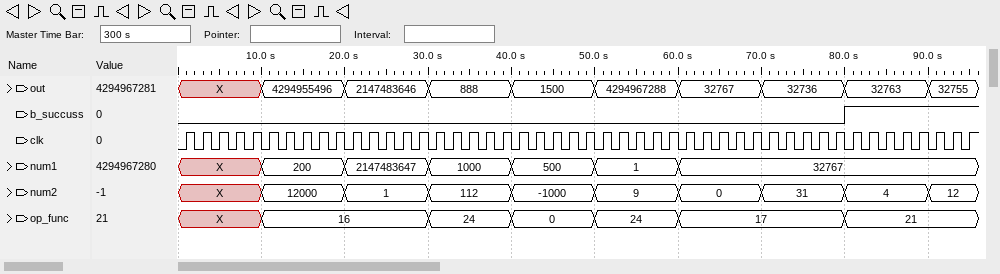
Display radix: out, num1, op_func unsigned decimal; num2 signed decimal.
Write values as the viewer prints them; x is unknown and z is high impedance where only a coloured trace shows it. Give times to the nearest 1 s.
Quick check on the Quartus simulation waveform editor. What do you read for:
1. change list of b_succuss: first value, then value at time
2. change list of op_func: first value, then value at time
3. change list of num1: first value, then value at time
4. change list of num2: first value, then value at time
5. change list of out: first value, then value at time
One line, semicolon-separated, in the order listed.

0, 1 at 80 s; X, 16 at 10 s, 24 at 30 s, 0 at 40 s, 24 at 50 s, 17 at 60 s, 21 at 80 s; X, 200 at 10 s, 2147483647 at 20 s, 1000 at 30 s, 500 at 40 s, 1 at 50 s, 32767 at 60 s; X, 12000 at 10 s, 1 at 20 s, 112 at 30 s, -1000 at 40 s, 9 at 50 s, 0 at 60 s, 31 at 70 s, 4 at 80 s, 12 at 90 s; X, 4294955496 at 10 s, 2147483646 at 20 s, 888 at 30 s, 1500 at 40 s, 4294967288 at 50 s, 32767 at 60 s, 32736 at 70 s, 32763 at 80 s, 32755 at 90 s
